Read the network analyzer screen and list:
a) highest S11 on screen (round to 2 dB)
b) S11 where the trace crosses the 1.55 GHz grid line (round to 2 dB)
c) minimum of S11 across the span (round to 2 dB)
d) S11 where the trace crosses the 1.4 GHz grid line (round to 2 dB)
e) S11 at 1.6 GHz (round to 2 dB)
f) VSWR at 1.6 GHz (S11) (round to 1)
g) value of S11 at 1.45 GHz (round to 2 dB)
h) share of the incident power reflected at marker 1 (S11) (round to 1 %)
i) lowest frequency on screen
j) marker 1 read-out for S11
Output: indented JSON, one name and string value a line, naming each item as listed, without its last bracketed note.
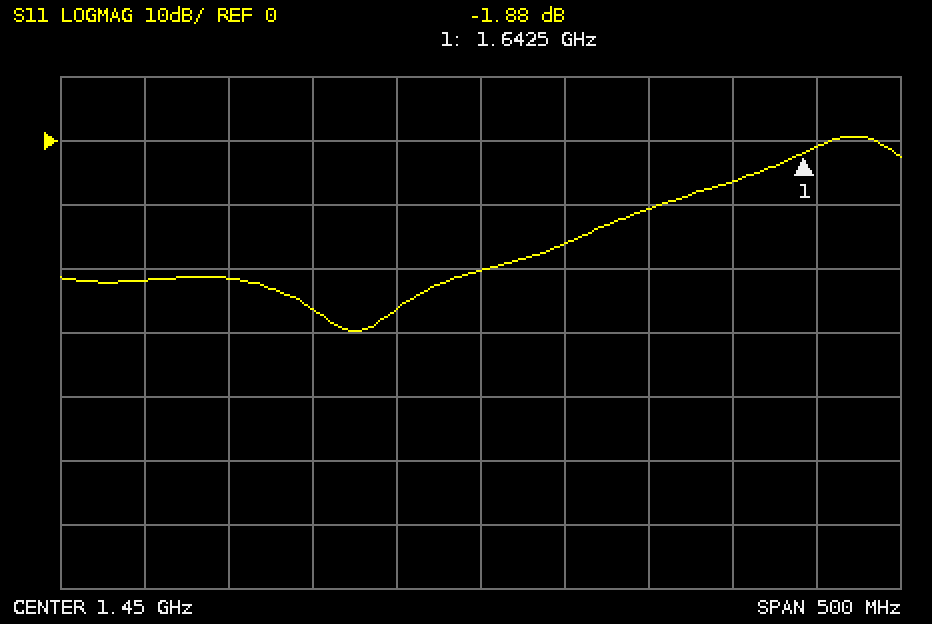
{
  "highest S11 on screen": "0 dB",
  "S11 where the trace crosses the 1.55 GHz grid line": "-10 dB",
  "minimum of S11 across the span": "-30 dB",
  "S11 where the trace crosses the 1.4 GHz grid line": "-26 dB",
  "S11 at 1.6 GHz": "-6 dB",
  "VSWR at 1.6 GHz (S11)": "3",
  "value of S11 at 1.45 GHz": "-20 dB",
  "share of the incident power reflected at marker 1 (S11)": "65 %",
  "lowest frequency on screen": "1.2 GHz",
  "marker 1 read-out for S11": "-1.88 dB"
}
